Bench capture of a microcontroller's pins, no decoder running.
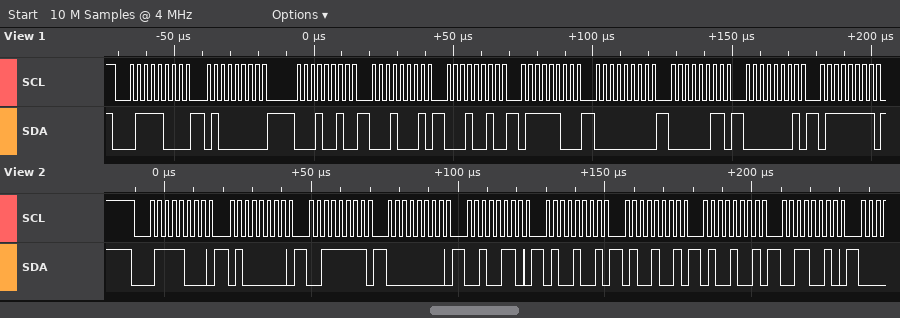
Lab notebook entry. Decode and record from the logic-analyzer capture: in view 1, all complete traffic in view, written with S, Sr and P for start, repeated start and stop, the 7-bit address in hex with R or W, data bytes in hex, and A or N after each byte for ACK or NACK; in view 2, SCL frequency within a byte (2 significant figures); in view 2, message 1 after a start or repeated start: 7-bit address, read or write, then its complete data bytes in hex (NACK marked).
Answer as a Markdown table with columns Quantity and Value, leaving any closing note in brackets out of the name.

| Quantity | Value |
|---|---|
| in view 1, all complete traffic in view, written with S, Sr and P for start, repeated start and stop, the 7-bit address in hex with R or W, data bytes in hex, and A or N after each byte for ACK or NACK | S 3CW A 40 A 12 A 11 A 12 A 7C A 00 A 03 A 01 A 7F A |
| in view 2, SCL frequency within a byte | 400 kHz |
| in view 2, message 1 after a start or repeated start: 7-bit address, read or write, then its complete data bytes in hex | 0x3C write: 40 3F 00 26 49 49 49 32 |
